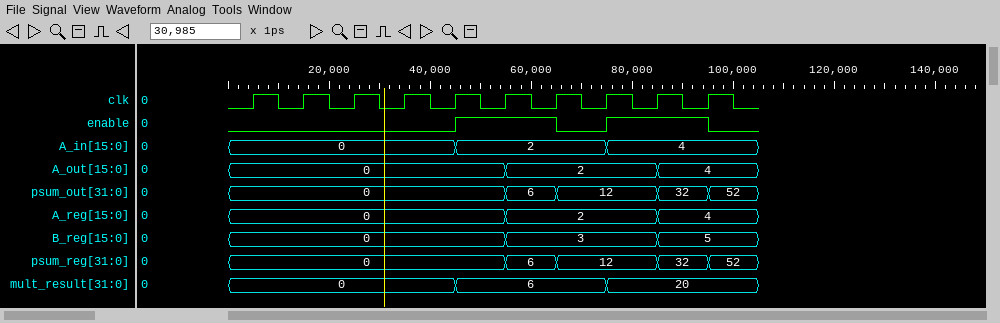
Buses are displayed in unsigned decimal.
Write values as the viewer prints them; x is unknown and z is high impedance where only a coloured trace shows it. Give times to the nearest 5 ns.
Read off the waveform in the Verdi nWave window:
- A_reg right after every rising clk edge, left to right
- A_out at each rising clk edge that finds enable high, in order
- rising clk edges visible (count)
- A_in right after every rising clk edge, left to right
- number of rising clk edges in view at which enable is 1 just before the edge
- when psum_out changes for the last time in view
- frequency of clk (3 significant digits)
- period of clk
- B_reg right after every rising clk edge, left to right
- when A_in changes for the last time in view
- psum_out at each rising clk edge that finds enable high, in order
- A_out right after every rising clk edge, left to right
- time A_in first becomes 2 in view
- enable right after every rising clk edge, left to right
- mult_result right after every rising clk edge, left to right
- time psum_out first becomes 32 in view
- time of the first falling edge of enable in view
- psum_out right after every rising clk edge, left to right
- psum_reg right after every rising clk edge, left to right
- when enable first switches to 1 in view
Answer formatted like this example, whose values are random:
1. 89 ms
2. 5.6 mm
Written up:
1. 0, 0, 0, 0, 0, 2, 2, 2, 4, 4
2. 0, 2, 2, 4
3. 10
4. 0, 0, 0, 0, 2, 2, 2, 4, 4, 4
5. 4
6. 95 ns
7. 100 MHz
8. 10 ns
9. 0, 0, 0, 0, 0, 3, 3, 3, 5, 5
10. 75 ns
11. 0, 6, 12, 32
12. 0, 0, 0, 0, 0, 2, 2, 2, 4, 4
13. 45 ns
14. 0 0 0 0 1 1 0 1 1 0
15. 0, 0, 0, 0, 6, 6, 6, 20, 20, 20
16. 85 ns
17. 65 ns
18. 0, 0, 0, 0, 0, 6, 12, 12, 32, 52
19. 0, 0, 0, 0, 0, 6, 12, 12, 32, 52
20. 45 ns
